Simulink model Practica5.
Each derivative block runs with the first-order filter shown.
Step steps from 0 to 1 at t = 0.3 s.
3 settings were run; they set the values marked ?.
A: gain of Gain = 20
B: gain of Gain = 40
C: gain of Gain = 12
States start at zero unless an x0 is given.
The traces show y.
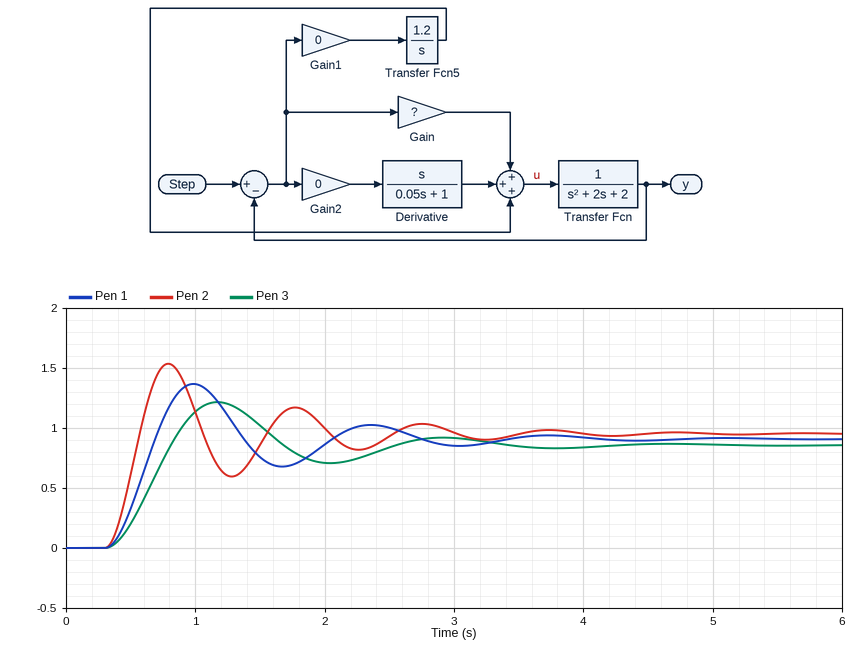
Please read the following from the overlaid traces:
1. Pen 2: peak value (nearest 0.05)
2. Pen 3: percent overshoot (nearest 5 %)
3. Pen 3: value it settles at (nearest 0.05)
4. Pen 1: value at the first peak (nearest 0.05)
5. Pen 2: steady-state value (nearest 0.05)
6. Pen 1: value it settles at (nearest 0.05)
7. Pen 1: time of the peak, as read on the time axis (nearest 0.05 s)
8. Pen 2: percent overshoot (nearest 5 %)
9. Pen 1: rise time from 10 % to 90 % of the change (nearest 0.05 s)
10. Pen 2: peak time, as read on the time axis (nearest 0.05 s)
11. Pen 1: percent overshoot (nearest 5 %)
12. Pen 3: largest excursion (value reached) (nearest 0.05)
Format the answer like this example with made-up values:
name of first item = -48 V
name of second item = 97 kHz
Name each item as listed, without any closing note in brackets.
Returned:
Pen 2: peak value = 1.55
Pen 3: percent overshoot = 40 %
Pen 3: value it settles at = 0.85
Pen 1: value at the first peak = 1.35
Pen 2: steady-state value = 0.95
Pen 1: value it settles at = 0.90
Pen 1: time of the peak, as read on the time axis = 1.00 s
Pen 2: percent overshoot = 60 %
Pen 1: rise time from 10 % to 90 % of the change = 0.25 s
Pen 2: peak time, as read on the time axis = 0.80 s
Pen 1: percent overshoot = 50 %
Pen 3: largest excursion (value reached) = 1.20
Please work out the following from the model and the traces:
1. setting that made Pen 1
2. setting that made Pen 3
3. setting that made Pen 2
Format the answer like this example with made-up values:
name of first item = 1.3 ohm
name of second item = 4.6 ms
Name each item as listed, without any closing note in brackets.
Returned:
setting that made Pen 1 = A
setting that made Pen 3 = C
setting that made Pen 2 = B
